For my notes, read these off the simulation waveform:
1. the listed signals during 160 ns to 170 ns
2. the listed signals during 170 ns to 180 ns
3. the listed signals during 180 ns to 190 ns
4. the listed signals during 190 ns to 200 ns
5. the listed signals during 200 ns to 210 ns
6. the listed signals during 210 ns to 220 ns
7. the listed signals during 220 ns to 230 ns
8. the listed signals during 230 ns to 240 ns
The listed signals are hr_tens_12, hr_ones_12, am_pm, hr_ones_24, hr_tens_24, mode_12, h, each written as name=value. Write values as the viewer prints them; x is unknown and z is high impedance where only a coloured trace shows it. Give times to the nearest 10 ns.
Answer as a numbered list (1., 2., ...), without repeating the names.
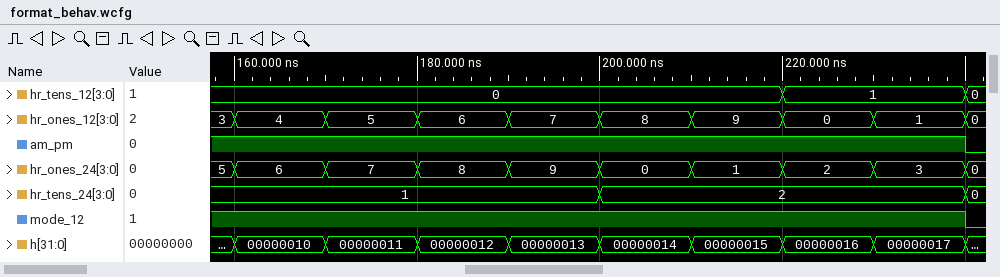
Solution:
1. hr_tens_12=0, hr_ones_12=4, am_pm=1, hr_ones_24=6, hr_tens_24=1, mode_12=1, h=00000010
2. hr_tens_12=0, hr_ones_12=5, am_pm=1, hr_ones_24=7, hr_tens_24=1, mode_12=1, h=00000011
3. hr_tens_12=0, hr_ones_12=6, am_pm=1, hr_ones_24=8, hr_tens_24=1, mode_12=1, h=00000012
4. hr_tens_12=0, hr_ones_12=7, am_pm=1, hr_ones_24=9, hr_tens_24=1, mode_12=1, h=00000013
5. hr_tens_12=0, hr_ones_12=8, am_pm=1, hr_ones_24=0, hr_tens_24=2, mode_12=1, h=00000014
6. hr_tens_12=0, hr_ones_12=9, am_pm=1, hr_ones_24=1, hr_tens_24=2, mode_12=1, h=00000015
7. hr_tens_12=1, hr_ones_12=0, am_pm=1, hr_ones_24=2, hr_tens_24=2, mode_12=1, h=00000016
8. hr_tens_12=1, hr_ones_12=1, am_pm=1, hr_ones_24=3, hr_tens_24=2, mode_12=1, h=00000017
